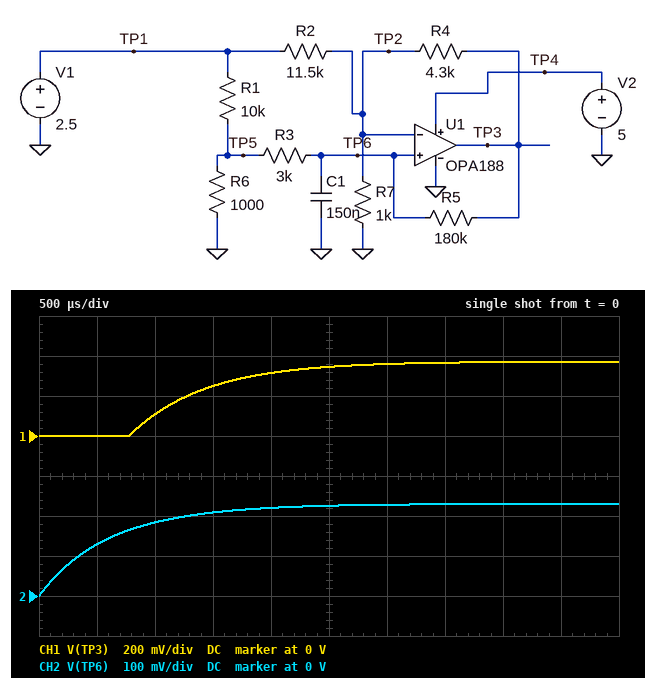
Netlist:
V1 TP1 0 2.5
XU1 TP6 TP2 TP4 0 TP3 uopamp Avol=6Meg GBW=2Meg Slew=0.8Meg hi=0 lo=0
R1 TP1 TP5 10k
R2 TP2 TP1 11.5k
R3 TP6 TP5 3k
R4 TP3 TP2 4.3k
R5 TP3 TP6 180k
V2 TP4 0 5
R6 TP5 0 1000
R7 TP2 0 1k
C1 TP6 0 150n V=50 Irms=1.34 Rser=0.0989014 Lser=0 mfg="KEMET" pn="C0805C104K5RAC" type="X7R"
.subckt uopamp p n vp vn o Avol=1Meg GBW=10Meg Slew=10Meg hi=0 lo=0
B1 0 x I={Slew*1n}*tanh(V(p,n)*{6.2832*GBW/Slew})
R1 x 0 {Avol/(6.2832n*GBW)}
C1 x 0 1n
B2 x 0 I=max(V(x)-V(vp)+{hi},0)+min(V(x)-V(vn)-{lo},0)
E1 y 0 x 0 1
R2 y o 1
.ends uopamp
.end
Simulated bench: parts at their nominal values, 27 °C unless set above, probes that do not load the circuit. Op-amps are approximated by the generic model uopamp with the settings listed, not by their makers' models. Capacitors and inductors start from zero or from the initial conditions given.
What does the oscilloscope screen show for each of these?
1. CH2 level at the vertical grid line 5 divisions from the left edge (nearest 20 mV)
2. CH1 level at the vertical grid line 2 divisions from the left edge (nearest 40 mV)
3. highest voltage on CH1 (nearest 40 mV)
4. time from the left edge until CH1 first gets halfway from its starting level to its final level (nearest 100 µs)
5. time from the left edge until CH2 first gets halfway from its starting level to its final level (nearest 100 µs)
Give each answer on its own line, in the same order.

220 mV
120 mV
360 mV
1.2 ms
400 µs
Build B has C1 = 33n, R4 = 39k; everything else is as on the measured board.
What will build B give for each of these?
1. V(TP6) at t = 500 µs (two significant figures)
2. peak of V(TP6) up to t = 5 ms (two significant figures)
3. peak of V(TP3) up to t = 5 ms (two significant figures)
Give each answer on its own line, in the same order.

240 mV
330 mV
5.0 V
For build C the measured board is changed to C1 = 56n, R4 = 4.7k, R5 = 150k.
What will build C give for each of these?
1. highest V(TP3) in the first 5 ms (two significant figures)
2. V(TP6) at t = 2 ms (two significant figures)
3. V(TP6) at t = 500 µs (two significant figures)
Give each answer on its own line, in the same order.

390 mV
230 mV
200 mV
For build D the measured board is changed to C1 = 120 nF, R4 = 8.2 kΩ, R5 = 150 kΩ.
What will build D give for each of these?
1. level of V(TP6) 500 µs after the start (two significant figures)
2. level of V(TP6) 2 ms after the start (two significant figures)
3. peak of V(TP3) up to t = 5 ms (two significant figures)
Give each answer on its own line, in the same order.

150 mV
230 mV
550 mV
